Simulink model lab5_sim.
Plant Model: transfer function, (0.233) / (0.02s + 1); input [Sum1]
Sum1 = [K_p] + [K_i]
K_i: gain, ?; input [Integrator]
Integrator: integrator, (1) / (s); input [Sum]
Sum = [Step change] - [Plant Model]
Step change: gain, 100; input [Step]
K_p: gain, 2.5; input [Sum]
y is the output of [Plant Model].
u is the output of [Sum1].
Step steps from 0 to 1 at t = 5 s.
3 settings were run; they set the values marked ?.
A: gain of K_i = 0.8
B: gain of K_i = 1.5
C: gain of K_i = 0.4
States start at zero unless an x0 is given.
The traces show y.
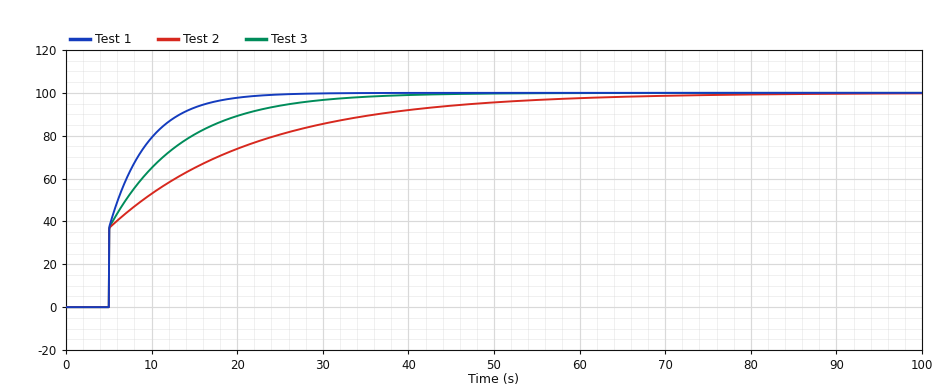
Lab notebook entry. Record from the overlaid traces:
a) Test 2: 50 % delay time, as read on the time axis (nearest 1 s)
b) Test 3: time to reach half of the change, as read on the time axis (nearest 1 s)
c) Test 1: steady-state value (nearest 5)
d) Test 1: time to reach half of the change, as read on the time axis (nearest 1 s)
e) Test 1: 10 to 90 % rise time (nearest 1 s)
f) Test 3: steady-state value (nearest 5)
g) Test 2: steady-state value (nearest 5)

9 s
7 s
100
6 s
8 s
100
100
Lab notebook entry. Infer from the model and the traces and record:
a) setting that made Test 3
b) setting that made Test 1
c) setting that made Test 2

A
B
C
